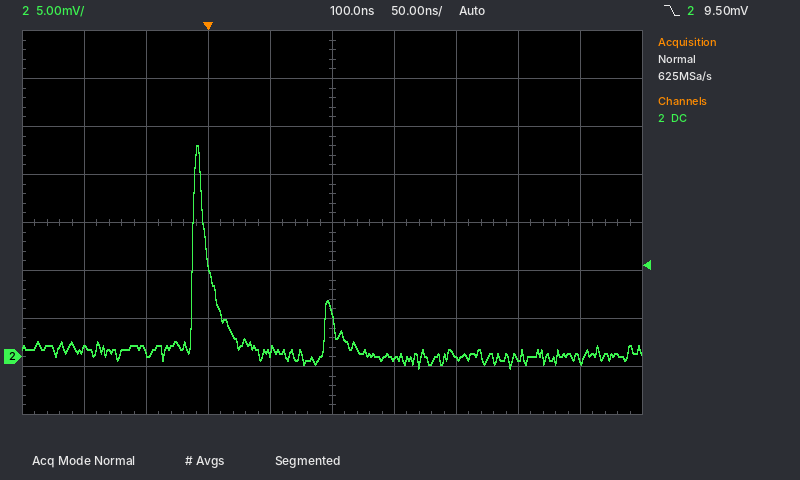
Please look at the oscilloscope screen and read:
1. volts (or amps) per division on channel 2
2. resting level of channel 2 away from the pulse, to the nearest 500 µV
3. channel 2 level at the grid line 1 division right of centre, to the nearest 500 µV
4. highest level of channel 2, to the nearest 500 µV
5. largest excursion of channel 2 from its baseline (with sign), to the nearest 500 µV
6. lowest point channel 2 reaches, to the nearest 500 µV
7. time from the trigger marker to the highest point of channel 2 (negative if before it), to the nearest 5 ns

5 mV
500 µV
0.0 mV
22.0 mV
+21.5 mV
-1.0 mV
-10 ns
